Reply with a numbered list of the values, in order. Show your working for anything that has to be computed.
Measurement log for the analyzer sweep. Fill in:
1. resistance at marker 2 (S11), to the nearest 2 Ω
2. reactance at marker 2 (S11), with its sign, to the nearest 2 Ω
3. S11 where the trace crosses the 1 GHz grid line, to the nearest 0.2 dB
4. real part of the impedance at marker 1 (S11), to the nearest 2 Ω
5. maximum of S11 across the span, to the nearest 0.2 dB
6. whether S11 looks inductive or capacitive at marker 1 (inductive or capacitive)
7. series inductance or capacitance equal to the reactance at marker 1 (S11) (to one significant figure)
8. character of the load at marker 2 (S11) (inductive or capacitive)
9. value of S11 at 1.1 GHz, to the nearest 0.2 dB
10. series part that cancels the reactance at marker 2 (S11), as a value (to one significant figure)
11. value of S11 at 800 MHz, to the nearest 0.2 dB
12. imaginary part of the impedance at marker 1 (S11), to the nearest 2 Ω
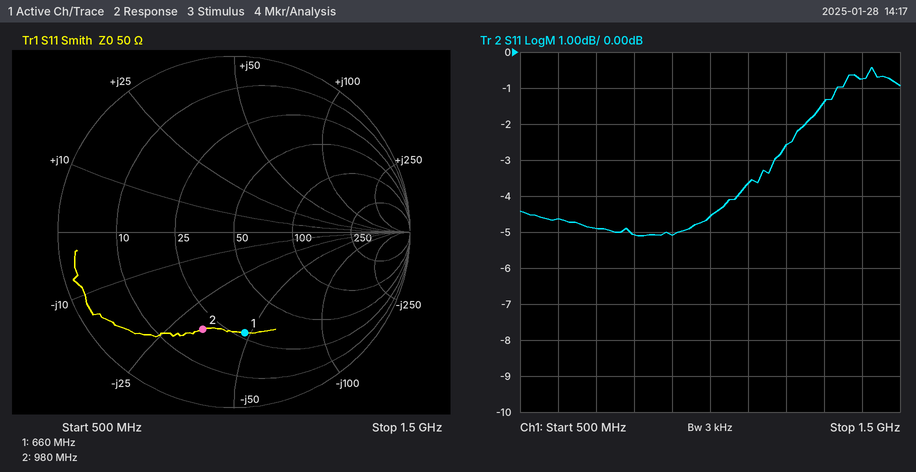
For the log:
1. 20 Ω
2. -32 Ω
3. -4.6 dB
4. 28 Ω
5. -0.4 dB
6. capacitive
7. C = 1/(2π × 660 MHz × 48 Ω) ≈ 5 pF
8. capacitive
9. -3.6 dB
10. L = 32 Ω/(2π × 980 MHz) ≈ 5 nH
11. -5.0 dB
12. -48 Ω
